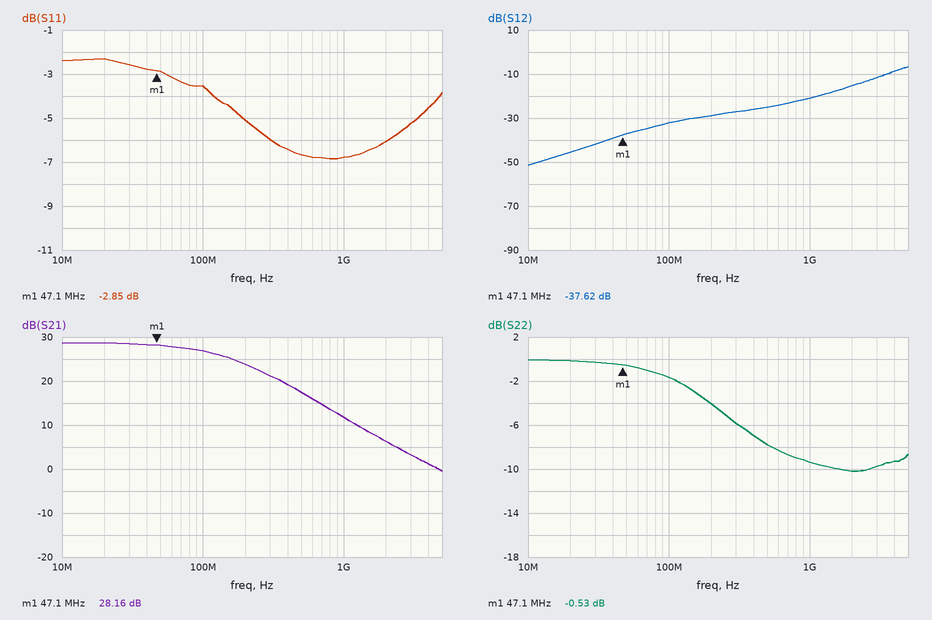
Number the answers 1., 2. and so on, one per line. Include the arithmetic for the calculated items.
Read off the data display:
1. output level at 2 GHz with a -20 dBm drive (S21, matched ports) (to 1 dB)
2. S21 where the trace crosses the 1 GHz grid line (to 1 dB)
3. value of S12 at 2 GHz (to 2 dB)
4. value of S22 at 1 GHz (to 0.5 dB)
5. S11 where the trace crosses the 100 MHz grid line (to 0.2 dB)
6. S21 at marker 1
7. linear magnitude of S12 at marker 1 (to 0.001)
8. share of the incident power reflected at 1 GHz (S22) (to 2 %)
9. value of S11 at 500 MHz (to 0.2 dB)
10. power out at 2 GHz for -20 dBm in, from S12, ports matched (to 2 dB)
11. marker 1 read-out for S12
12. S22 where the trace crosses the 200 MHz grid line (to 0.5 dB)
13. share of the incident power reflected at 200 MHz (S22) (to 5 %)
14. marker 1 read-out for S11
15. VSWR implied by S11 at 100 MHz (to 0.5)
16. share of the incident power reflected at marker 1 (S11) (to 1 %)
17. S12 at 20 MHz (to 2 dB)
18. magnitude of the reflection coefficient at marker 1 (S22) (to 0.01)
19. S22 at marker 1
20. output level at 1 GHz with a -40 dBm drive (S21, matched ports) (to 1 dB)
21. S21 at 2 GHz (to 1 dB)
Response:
1. -20 dBm + (6 dB) = -14 dBm
2. 12 dB
3. -16 dB
4. -9.5 dB
5. -3.6 dB
6. 28.16 dB
7. 10^(-37.62/20) ≈ 0.013
8. 10^(-9.5/10) ≈ 11.2 %, so 12 % to the nearest 2 %
9. -6.6 dB
10. -20 dBm + (-16 dB) = -36 dBm
11. -37.62 dB
12. -4.0 dB
13. 10^(-4/10) ≈ 40 %
14. -2.85 dB
15. |Γ| = 10^(-3.6/20) = 0.6607; VSWR = (1 + 0.6607)/(1 − 0.6607) ≈ 4.89, so 5.0 to the nearest 0.5
16. 10^(-2.85/10) ≈ 52 %
17. -46 dB
18. 10^(-0.53/20) ≈ 0.94
19. -0.53 dB
20. -40 dBm + (12 dB) = -28 dBm
21. 6 dB
